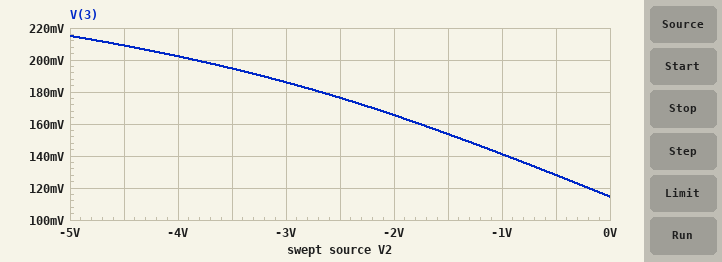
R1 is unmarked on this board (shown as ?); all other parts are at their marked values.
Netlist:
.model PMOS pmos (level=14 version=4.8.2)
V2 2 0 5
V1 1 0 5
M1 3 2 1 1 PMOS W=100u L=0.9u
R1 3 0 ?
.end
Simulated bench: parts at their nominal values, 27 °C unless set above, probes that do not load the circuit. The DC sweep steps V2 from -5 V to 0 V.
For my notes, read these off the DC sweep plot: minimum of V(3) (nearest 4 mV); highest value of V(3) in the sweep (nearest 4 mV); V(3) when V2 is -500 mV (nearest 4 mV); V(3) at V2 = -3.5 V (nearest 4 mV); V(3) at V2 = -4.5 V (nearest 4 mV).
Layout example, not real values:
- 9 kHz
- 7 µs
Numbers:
- 116 mV
- 216 mV
- 128 mV
- 196 mV
- 208 mV
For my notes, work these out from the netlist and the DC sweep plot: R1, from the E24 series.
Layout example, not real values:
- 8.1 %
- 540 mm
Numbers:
- 1.3 Ω
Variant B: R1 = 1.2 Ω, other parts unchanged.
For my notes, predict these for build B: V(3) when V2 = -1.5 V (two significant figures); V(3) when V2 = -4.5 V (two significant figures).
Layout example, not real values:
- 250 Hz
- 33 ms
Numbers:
- 140 mV
- 190 mV
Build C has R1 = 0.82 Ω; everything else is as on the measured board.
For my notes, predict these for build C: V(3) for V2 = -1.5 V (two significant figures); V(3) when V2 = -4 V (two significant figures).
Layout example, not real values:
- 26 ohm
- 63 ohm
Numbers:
- 97 mV
- 130 mV
